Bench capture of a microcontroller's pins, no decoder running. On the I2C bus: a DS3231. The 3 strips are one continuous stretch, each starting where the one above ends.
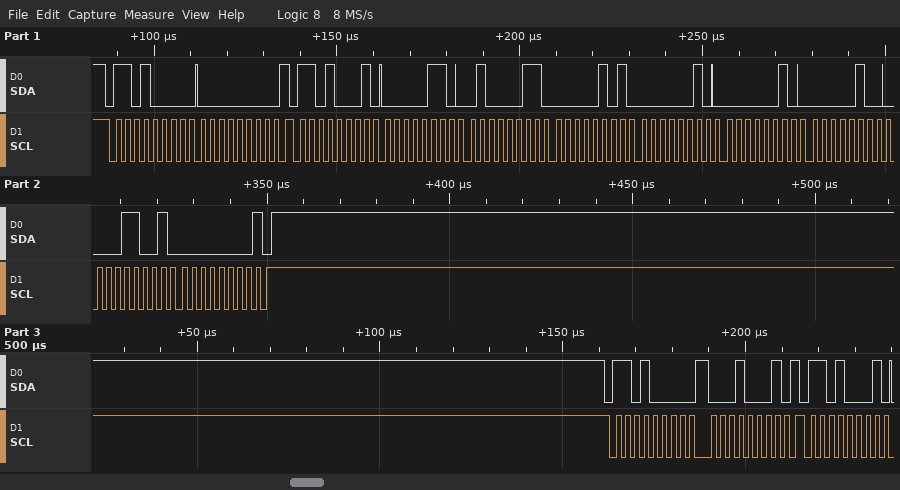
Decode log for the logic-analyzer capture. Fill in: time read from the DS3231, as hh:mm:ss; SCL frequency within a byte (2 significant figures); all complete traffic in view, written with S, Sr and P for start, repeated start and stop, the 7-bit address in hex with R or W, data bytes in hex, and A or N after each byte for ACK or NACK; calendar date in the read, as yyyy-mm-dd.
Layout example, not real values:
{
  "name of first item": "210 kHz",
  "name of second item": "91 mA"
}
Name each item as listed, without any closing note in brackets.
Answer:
{
  "time read from the DS3231, as hh:mm:ss": "05:43:06",
  "SCL frequency within a byte": "400 kHz",
  "all complete traffic in view, written with S, Sr and P for start, repeated start and stop, the 7-bit address in hex with R or W, data bytes in hex, and A or N after each byte for ACK or NACK": "S 68W A 00 A Sr 68R A 06 A 43 A 05 A 02 A 02 A 04 A 19 A 00 N P S 68W A 11 A Sr 68R A",
  "calendar date in the read, as yyyy-mm-dd": "2019-04-02"
}
